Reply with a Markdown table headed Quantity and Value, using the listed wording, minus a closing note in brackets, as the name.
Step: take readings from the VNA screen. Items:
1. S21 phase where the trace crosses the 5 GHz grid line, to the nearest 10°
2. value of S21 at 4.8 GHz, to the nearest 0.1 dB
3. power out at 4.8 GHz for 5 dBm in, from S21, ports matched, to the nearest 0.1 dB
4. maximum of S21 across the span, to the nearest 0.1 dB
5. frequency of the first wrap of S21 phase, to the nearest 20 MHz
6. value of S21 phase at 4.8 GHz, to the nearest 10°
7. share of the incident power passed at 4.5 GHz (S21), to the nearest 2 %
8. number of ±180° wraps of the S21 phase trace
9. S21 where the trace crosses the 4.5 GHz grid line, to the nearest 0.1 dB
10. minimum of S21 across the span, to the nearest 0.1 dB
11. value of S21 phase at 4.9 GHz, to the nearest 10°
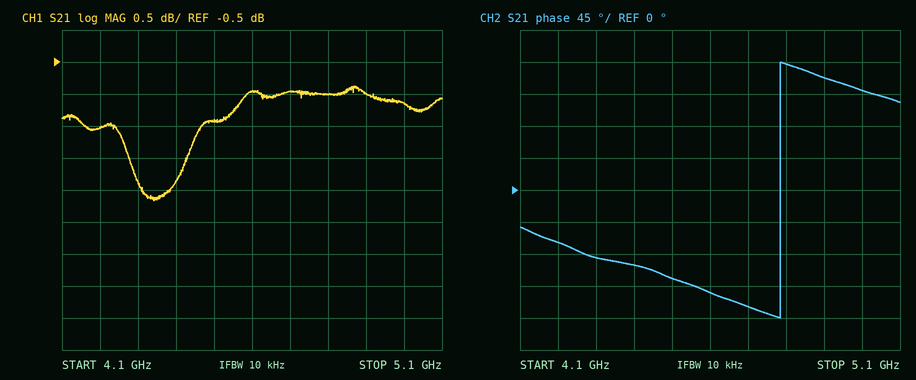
| Quantity | Value |
|---|---|
| S21 phase where the trace crosses the 5 GHz grid line, to the nearest 10° | 140° |
| value of S21 at 4.8 GHz, to the nearest 0.1 dB | -1.0 dB |
| power out at 4.8 GHz for 5 dBm in, from S21, ports matched, to the nearest 0.1 dB | 4.0 dBm |
| maximum of S21 across the span, to the nearest 0.1 dB | -0.9 dB |
| frequency of the first wrap of S21 phase, to the nearest 20 MHz | 4.78 GHz |
| value of S21 phase at 4.8 GHz, to the nearest 10° | 180° |
| share of the incident power passed at 4.5 GHz (S21), to the nearest 2 % | 72 % |
| number of ±180° wraps of the S21 phase trace | 1 |
| S21 where the trace crosses the 4.5 GHz grid line, to the nearest 0.1 dB | -1.4 dB |
| minimum of S21 across the span, to the nearest 0.1 dB | -2.7 dB |
| value of S21 phase at 4.9 GHz, to the nearest 10° | 160° |
